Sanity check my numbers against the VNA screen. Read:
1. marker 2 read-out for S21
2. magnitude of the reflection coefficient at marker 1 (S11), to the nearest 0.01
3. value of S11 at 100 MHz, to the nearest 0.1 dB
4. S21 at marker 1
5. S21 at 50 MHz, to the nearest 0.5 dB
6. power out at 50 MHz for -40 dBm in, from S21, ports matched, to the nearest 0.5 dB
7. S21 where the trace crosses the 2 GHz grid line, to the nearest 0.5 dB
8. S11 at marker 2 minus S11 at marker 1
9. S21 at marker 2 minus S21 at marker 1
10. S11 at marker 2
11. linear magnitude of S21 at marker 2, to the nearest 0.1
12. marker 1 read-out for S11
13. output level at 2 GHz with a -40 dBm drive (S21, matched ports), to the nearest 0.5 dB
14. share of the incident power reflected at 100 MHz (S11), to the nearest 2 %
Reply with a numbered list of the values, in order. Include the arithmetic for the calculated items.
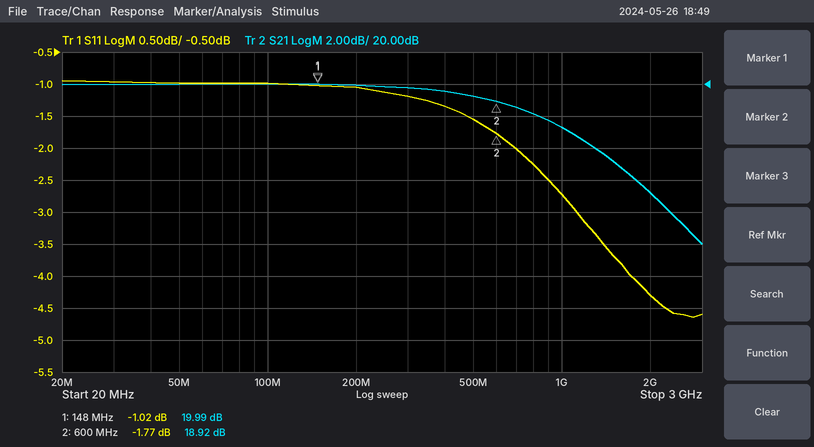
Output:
1. 18.92 dB
2. 10^(-1.02/20) ≈ 0.89
3. -1.0 dB
4. 19.99 dB
5. 20.0 dB
6. -40 dBm + (20.0 dB) = -20.0 dBm
7. 13.0 dB
8. -1.77 − (-1.02) = -0.75 dB
9. 18.92 − (19.99) = -1.07 dB
10. -1.77 dB
11. 10^(18.92/20) ≈ 8.8
12. -1.02 dB
13. -40 dBm + (13.0 dB) = -27.0 dBm
14. 10^(-1/10) ≈ 79.4 %, so 80 % to the nearest 2 %
